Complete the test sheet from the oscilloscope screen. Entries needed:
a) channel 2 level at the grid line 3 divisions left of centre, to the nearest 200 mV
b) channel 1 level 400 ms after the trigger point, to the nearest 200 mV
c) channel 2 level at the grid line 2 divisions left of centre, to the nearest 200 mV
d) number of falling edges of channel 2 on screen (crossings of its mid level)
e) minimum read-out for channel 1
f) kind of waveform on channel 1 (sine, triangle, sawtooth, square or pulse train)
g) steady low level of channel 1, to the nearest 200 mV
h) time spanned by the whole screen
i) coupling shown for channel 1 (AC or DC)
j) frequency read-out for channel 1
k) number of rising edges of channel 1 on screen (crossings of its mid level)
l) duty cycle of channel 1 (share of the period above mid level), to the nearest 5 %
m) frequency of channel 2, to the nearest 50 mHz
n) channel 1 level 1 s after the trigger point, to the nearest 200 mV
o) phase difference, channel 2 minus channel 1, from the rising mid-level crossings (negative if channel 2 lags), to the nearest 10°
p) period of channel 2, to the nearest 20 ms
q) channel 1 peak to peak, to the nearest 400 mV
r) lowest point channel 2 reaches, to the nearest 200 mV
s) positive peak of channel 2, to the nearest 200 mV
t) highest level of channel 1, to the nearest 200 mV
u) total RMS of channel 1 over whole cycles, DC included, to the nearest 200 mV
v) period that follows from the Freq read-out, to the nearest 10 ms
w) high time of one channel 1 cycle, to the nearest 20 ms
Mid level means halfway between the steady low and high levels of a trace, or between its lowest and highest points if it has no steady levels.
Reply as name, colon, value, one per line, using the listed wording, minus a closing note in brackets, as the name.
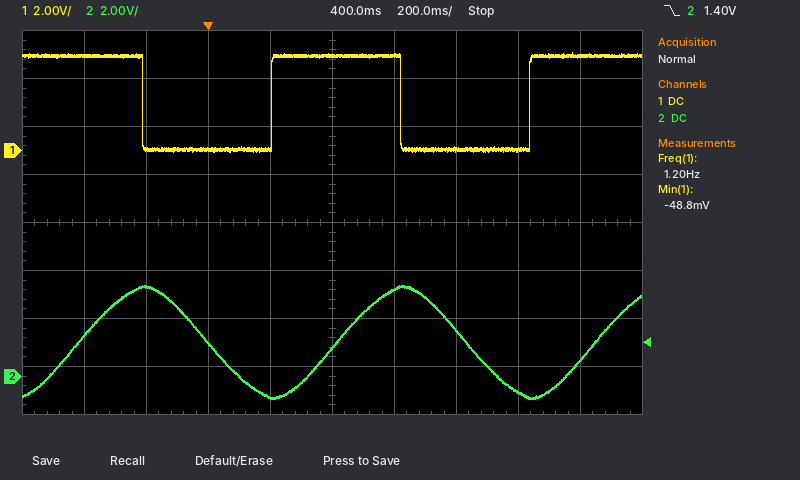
channel 2 level at the grid line 3 divisions left of centre, to the nearest 200 mV: 3.8 V
channel 1 level 400 ms after the trigger point, to the nearest 200 mV: 4.0 V
channel 2 level at the grid line 2 divisions left of centre, to the nearest 200 mV: 1.4 V
number of falling edges of channel 2 on screen: 2
minimum read-out for channel 1: -48.8 mV
kind of waveform on channel 1: square
steady low level of channel 1, to the nearest 200 mV: 0.0 V
time spanned by the whole screen: 2 s
coupling shown for channel 1: DC
frequency read-out for channel 1: 1.20 Hz
number of rising edges of channel 1 on screen: 2
duty cycle of channel 1 (share of the period above mid level), to the nearest 5 %: 50 %
frequency of channel 2, to the nearest 50 mHz: 1.20 Hz
channel 1 level 1 s after the trigger point, to the nearest 200 mV: 0.0 V
phase difference, channel 2 minus channel 1, from the rising mid-level crossings (negative if channel 2 lags), to the nearest 10°: -90°
period of channel 2, to the nearest 20 ms: 840 ms
channel 1 peak to peak, to the nearest 400 mV: 4.0 V
lowest point channel 2 reaches, to the nearest 200 mV: -1.0 V
positive peak of channel 2, to the nearest 200 mV: 3.8 V
highest level of channel 1, to the nearest 200 mV: 4.0 V
total RMS of channel 1 over whole cycles, DC included, to the nearest 200 mV: 2.8 V
period that follows from the Freq read-out, to the nearest 10 ms: 830 ms
high time of one channel 1 cycle, to the nearest 20 ms: 420 ms
